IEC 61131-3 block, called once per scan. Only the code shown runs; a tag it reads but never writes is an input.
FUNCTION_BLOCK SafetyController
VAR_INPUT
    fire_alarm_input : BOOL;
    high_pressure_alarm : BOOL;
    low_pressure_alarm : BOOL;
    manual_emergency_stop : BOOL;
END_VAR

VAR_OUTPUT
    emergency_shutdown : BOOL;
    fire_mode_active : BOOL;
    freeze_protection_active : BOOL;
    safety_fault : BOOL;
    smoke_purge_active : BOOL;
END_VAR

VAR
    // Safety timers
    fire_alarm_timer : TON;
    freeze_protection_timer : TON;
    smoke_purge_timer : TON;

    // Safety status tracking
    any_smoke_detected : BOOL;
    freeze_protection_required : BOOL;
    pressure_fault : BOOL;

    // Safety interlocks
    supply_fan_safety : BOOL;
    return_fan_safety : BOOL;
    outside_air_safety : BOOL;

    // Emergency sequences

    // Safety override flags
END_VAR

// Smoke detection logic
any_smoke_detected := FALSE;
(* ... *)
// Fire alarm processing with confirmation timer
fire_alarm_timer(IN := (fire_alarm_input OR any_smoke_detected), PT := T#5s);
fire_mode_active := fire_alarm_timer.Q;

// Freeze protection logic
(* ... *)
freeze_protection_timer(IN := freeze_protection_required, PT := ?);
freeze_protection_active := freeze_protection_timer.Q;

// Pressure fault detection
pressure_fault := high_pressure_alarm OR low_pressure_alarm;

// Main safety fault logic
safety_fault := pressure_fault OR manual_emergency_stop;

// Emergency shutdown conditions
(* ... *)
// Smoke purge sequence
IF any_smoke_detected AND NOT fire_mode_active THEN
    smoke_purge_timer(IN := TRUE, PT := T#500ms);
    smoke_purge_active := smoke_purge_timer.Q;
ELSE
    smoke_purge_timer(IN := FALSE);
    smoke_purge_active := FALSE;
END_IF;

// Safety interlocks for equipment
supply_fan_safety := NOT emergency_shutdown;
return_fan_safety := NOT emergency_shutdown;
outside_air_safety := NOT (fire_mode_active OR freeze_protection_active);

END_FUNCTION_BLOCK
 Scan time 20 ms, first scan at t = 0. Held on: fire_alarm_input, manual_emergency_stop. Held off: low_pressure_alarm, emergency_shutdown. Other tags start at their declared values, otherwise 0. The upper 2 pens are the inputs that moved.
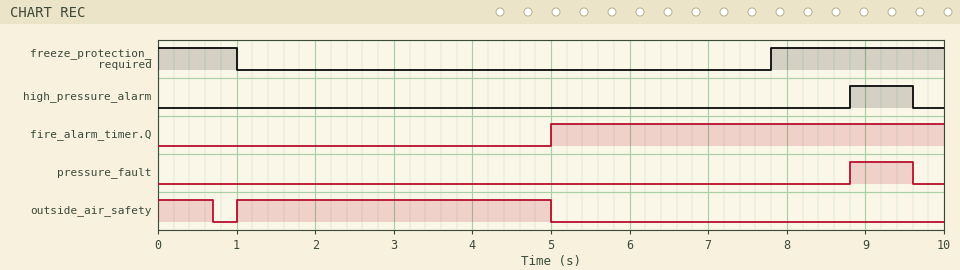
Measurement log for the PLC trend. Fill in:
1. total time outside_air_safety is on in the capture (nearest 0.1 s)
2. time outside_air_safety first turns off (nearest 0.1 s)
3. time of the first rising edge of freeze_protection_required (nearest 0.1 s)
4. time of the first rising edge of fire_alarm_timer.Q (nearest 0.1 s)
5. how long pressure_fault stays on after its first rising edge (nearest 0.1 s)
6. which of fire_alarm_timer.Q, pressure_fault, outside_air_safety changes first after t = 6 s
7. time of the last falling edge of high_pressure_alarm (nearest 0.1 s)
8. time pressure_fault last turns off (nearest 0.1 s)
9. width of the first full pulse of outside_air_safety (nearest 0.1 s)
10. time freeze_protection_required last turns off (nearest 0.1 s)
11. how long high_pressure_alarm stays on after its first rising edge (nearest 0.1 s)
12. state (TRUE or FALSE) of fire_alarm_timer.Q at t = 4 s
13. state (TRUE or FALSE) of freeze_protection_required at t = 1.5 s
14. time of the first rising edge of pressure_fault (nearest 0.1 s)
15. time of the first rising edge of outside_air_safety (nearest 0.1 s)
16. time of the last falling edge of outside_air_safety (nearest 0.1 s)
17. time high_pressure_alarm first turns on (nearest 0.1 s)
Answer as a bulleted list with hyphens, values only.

- 4.7 s
- 0.7 s
- 7.8 s
- 5.0 s
- 0.8 s
- pressure_fault
- 9.6 s
- 9.6 s
- 4.0 s
- 1.0 s
- 0.8 s
- FALSE
- FALSE
- 8.8 s
- 1.0 s
- 5.0 s
- 8.8 s
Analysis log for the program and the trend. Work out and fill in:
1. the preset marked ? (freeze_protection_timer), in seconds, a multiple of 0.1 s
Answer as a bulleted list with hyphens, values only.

- 0.7 s
